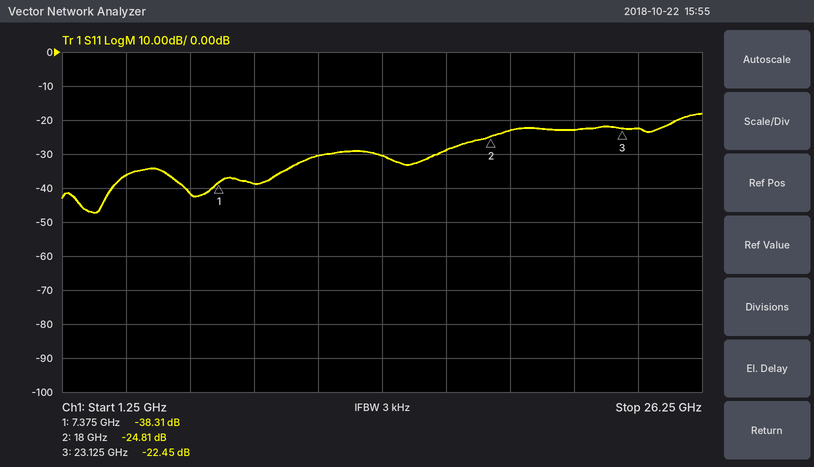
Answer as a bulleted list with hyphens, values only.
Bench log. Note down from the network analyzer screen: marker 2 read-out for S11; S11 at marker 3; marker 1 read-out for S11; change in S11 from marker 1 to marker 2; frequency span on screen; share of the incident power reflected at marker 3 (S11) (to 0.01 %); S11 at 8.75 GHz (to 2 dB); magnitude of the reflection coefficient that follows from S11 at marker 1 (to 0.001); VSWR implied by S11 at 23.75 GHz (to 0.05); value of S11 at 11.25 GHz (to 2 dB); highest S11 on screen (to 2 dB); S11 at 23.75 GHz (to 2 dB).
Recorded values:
- -24.81 dB
- -22.45 dB
- -38.31 dB
- 13.50 dB
- 25 GHz
- 0.57 %
- -38 dB
- 0.012
- 1.15
- -30 dB
- -18 dB
- -22 dB
